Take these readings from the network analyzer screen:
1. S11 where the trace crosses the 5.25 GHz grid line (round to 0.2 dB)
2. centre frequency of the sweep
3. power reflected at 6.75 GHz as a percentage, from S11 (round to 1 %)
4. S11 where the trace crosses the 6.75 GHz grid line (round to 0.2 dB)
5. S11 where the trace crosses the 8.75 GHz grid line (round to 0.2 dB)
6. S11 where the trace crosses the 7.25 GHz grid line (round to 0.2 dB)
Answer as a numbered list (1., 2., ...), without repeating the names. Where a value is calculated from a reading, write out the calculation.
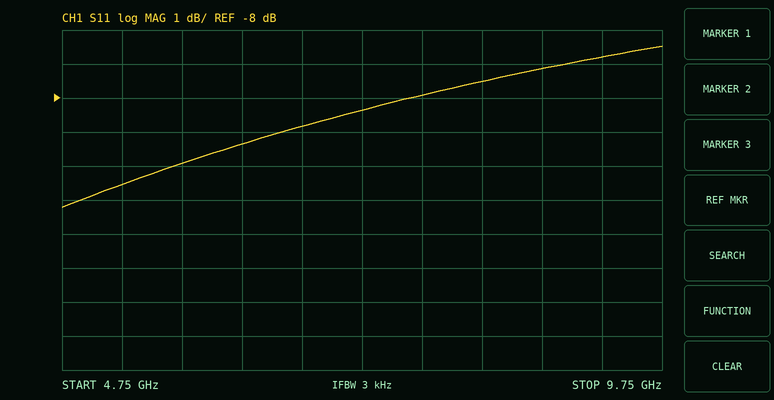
1. -10.6 dB
2. 7.25 GHz
3. 10^(-8.8/10) ≈ 13 %
4. -8.8 dB
5. -7.2 dB
6. -8.4 dB
